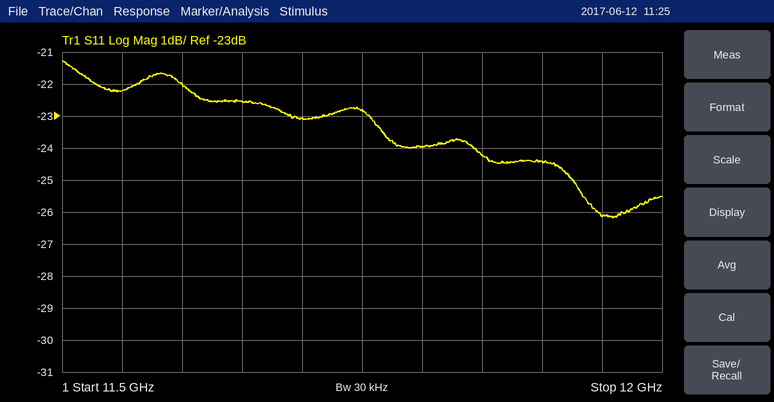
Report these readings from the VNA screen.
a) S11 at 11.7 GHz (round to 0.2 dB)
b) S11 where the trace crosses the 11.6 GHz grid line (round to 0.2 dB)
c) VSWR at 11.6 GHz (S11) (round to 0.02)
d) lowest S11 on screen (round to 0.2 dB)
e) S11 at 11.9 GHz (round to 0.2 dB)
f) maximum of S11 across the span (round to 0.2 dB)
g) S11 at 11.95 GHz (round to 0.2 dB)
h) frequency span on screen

-23.0 dB
-22.0 dB
1.18
-26.2 dB
-24.4 dB
-21.2 dB
-26.2 dB
500 MHz
